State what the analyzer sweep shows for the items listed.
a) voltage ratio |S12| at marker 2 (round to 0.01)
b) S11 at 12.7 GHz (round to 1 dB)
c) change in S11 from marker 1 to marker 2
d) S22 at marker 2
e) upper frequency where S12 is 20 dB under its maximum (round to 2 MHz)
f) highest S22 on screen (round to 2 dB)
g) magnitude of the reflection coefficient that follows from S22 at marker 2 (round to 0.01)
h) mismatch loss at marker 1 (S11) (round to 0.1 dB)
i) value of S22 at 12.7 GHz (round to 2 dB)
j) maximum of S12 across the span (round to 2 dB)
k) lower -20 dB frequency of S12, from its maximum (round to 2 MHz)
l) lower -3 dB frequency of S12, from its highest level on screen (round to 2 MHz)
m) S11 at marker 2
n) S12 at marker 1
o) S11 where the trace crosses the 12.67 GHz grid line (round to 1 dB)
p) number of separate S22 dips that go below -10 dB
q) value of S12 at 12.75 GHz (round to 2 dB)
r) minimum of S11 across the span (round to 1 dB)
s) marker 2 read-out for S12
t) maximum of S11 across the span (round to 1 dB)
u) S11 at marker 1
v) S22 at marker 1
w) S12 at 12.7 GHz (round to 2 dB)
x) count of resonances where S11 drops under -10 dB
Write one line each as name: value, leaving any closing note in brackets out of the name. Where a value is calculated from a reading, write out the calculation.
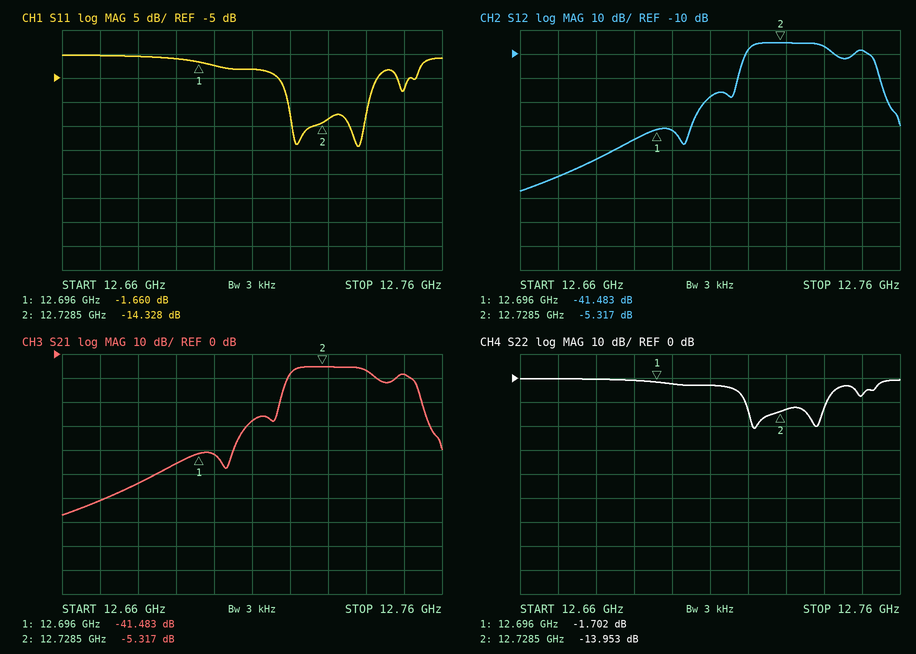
voltage ratio |S12| at marker 2: 10^(-5.317/20) ≈ 0.54
S11 at 12.7 GHz: -2 dB
change in S11 from marker 1 to marker 2: -14.328 − (-1.66) = -12.668 dB
S22 at marker 2: -13.953 dB
upper frequency where S12 is 20 dB under its maximum: 12.756 GHz
highest S22 on screen: 0 dB
magnitude of the reflection coefficient that follows from S22 at marker 2: 10^(-13.953/20) ≈ 0.20
mismatch loss at marker 1 (S11): −10 log10(1 − 10^(-1.66/10)) ≈ 5.0 dB
value of S22 at 12.7 GHz: -2 dB
maximum of S12 across the span: -6 dB
lower -20 dB frequency of S12, from its maximum: 12.716 GHz
lower -3 dB frequency of S12, from its highest level on screen: 12.720 GHz
S11 at marker 2: -14.328 dB
S12 at marker 1: -41.483 dB
S11 where the trace crosses the 12.67 GHz grid line: 0 dB
number of separate S22 dips that go below -10 dB: 2
value of S12 at 12.75 GHz: -8 dB
minimum of S11 across the span: -19 dB
marker 2 read-out for S12: -5.317 dB
maximum of S11 across the span: 0 dB
S11 at marker 1: -1.660 dB
S22 at marker 1: -1.702 dB
S12 at 12.7 GHz: -42 dB
count of resonances where S11 drops under -10 dB: 2
